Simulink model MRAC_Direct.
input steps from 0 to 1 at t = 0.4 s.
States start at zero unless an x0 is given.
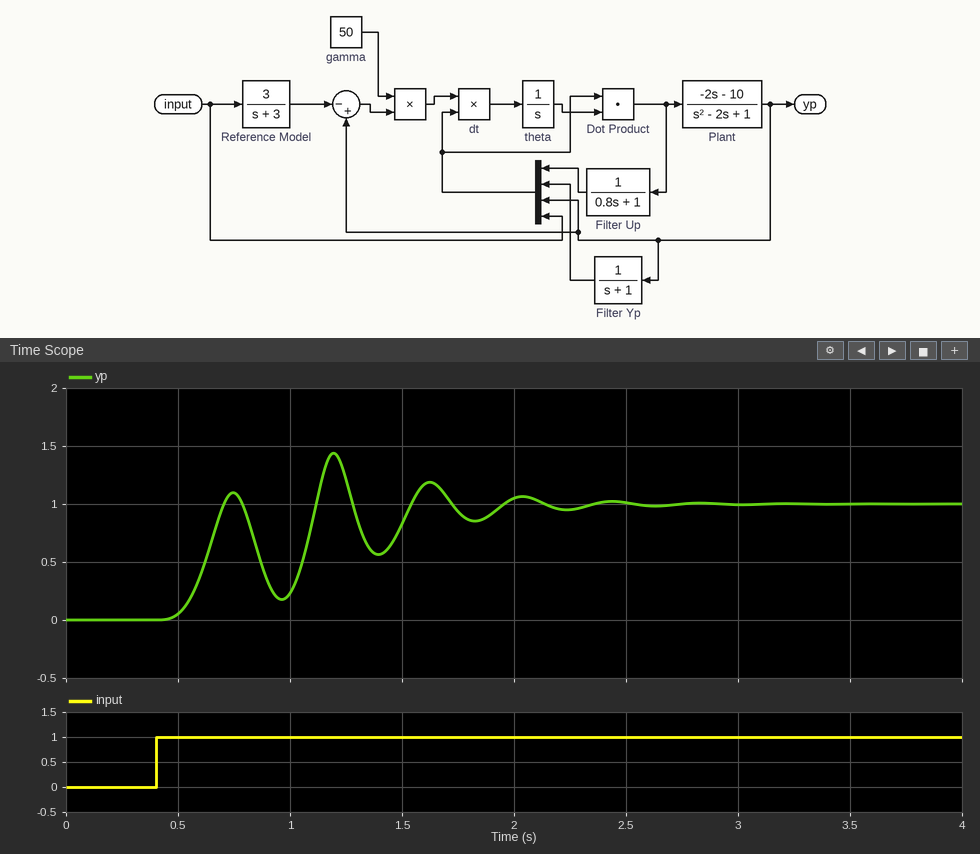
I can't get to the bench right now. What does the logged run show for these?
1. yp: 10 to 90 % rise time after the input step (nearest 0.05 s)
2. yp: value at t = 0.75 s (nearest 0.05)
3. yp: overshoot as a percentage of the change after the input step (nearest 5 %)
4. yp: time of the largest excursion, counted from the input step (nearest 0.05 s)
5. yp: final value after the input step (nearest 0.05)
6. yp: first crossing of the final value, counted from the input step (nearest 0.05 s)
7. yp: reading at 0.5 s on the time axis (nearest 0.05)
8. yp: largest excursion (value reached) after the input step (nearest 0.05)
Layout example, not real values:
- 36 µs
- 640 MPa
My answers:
- 0.15 s
- 1.10
- 45 %
- 0.80 s
- 1.00
- 0.30 s
- 0.05
- 1.45
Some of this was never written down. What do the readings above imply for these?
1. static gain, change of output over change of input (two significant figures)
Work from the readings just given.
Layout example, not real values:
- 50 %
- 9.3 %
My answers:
- 1.0
